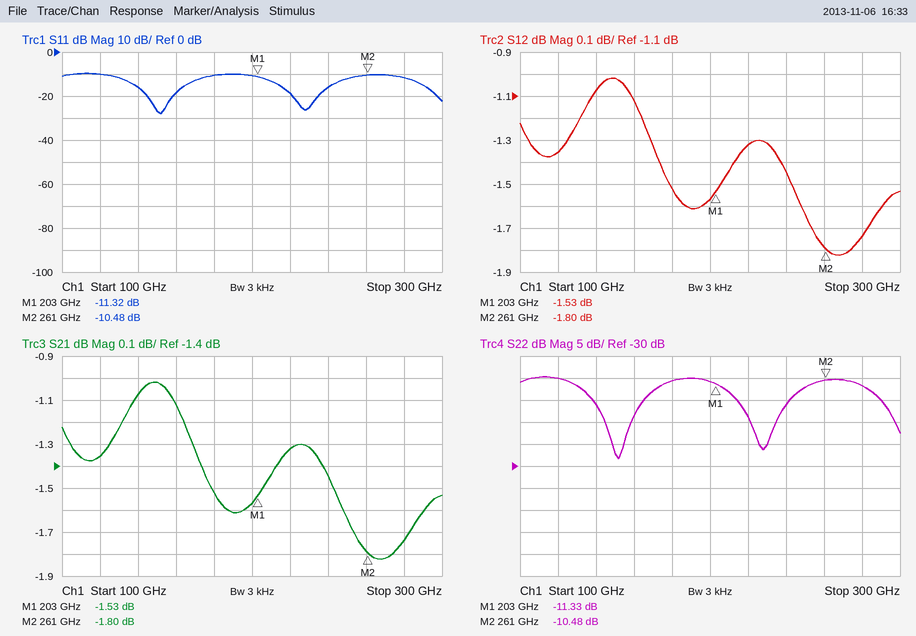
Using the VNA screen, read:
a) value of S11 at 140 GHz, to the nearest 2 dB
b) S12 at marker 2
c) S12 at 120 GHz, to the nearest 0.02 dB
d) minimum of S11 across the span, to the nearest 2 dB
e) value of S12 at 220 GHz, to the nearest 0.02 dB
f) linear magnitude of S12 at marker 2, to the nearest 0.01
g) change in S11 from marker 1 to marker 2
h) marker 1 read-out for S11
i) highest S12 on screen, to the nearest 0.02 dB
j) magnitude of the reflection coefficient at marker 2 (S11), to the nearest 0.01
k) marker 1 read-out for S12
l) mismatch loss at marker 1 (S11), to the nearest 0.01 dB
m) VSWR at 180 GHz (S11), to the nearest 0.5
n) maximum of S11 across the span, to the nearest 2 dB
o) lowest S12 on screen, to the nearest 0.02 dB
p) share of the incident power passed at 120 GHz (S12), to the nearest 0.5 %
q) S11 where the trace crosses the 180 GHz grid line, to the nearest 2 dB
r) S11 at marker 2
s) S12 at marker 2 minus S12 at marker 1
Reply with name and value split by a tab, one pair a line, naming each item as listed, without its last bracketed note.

value of S11 at 140 GHz, to the nearest 2 dB	-16 dB
S12 at marker 2	-1.80 dB
S12 at 120 GHz, to the nearest 0.02 dB	-1.36 dB
minimum of S11 across the span, to the nearest 2 dB	-28 dB
value of S12 at 220 GHz, to the nearest 0.02 dB	-1.32 dB
linear magnitude of S12 at marker 2, to the nearest 0.01	0.81
change in S11 from marker 1 to marker 2	0.84 dB
marker 1 read-out for S11	-11.32 dB
highest S12 on screen, to the nearest 0.02 dB	-1.02 dB
magnitude of the reflection coefficient at marker 2 (S11), to the nearest 0.01	0.30
marker 1 read-out for S12	-1.53 dB
mismatch loss at marker 1 (S11), to the nearest 0.01 dB	0.33 dB
VSWR at 180 GHz (S11), to the nearest 0.5	2.0
maximum of S11 across the span, to the nearest 2 dB	-10 dB
lowest S12 on screen, to the nearest 0.02 dB	-1.82 dB
share of the incident power passed at 120 GHz (S12), to the nearest 0.5 %	73.0 %
S11 where the trace crosses the 180 GHz grid line, to the nearest 2 dB	-10 dB
S11 at marker 2	-10.48 dB
S12 at marker 2 minus S12 at marker 1	-0.27 dB
